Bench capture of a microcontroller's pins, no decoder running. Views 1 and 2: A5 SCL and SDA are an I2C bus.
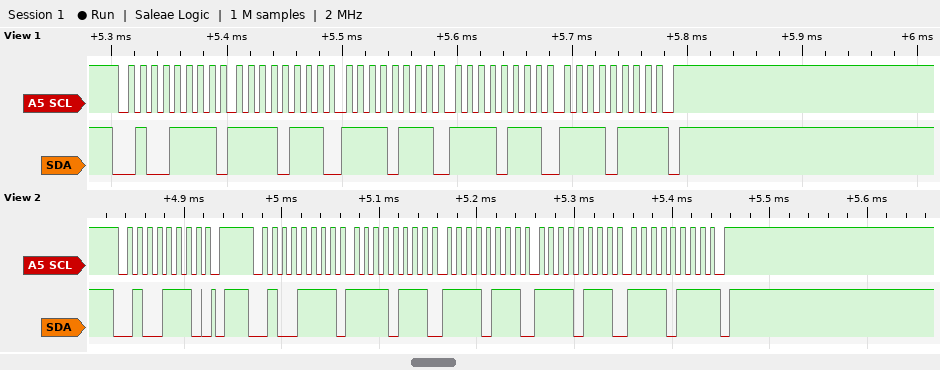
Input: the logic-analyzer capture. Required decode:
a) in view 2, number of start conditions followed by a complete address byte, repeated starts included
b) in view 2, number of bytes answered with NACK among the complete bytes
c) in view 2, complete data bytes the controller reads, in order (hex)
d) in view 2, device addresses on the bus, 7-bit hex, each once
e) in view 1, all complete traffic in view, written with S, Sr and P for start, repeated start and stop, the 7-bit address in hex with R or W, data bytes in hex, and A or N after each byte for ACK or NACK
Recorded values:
2
1
F7 F7 F7 F7
0x27
S 27R A F7 A F7 A F7 A F7 N P
